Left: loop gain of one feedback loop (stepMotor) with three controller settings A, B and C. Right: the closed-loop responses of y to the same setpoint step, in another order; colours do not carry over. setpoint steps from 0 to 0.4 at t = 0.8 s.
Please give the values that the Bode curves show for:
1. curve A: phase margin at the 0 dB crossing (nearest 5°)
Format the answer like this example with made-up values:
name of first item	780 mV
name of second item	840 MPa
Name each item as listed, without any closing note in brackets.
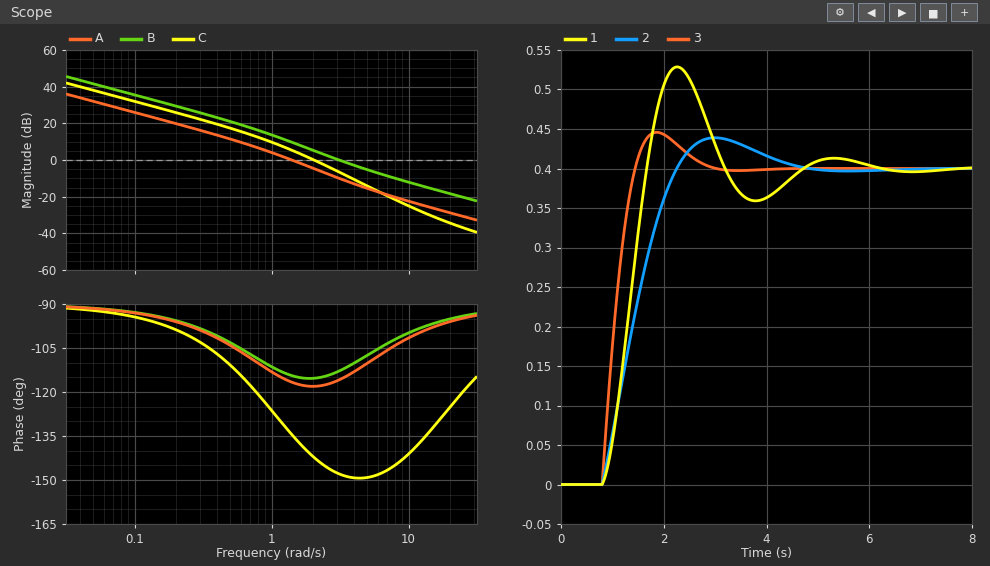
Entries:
curve A: phase margin at the 0 dB crossing	65°
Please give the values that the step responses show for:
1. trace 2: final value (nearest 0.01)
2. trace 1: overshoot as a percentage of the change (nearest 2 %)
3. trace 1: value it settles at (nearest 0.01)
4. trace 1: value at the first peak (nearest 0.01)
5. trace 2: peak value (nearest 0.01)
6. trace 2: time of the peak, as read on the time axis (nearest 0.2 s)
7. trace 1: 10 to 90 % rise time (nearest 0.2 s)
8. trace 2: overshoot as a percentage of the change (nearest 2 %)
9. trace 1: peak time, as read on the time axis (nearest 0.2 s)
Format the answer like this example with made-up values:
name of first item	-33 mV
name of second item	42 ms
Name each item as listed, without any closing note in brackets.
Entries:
trace 2: final value	0.40
trace 1: overshoot as a percentage of the change	32 %
trace 1: value it settles at	0.40
trace 1: value at the first peak	0.53
trace 2: peak value	0.44
trace 2: time of the peak, as read on the time axis	3.0 s
trace 1: 10 to 90 % rise time	0.6 s
trace 2: overshoot as a percentage of the change	10 %
trace 1: peak time, as read on the time axis	2.2 s
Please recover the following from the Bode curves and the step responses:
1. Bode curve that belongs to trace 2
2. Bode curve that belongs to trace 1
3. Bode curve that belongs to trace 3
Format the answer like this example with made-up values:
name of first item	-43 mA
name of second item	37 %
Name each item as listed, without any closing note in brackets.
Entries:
Bode curve that belongs to trace 2	A
Bode curve that belongs to trace 1	C
Bode curve that belongs to trace 3	B
